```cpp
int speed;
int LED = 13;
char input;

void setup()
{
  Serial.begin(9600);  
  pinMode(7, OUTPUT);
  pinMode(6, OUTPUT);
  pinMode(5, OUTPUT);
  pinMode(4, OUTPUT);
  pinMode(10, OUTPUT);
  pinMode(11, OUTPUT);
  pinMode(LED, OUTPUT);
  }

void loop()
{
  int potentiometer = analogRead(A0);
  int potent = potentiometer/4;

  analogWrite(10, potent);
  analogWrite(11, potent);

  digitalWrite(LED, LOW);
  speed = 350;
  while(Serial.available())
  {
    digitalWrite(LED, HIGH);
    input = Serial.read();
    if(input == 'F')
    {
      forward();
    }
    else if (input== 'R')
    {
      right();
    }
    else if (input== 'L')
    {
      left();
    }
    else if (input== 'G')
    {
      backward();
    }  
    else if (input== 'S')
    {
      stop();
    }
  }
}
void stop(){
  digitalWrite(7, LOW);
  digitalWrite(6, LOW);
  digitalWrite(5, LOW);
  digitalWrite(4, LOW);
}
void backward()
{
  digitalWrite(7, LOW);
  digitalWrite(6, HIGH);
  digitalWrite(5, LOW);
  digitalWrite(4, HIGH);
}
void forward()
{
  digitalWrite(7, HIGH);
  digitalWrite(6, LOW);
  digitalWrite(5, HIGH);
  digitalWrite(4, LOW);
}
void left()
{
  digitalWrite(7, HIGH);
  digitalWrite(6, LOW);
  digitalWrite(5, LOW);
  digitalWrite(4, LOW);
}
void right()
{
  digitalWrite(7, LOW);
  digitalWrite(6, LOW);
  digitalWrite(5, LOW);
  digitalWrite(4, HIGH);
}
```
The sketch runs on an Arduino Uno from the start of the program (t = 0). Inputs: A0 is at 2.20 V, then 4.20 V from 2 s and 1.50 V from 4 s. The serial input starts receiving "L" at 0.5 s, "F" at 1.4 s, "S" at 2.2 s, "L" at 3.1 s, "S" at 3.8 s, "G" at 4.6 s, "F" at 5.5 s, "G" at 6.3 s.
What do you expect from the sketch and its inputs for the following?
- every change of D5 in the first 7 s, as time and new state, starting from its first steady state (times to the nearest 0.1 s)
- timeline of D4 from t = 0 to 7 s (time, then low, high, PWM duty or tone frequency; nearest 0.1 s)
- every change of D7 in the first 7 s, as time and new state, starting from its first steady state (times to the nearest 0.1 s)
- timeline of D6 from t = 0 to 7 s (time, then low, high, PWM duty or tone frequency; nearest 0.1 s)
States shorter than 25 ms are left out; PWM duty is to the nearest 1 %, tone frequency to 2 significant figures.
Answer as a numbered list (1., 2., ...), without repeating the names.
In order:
1. 0 s low; 1.4 s high; 2.2 s low; 5.5 s high; 6.3 s low
2. 0 s low; 4.6 s high; 5.5 s low; 6.3 s high
3. 0 s low; 0.5 s high; 2.2 s low; 3.1 s high; 3.8 s low; 5.5 s high; 6.3 s low
4. 0 s low; 4.6 s high; 5.5 s low; 6.3 s high
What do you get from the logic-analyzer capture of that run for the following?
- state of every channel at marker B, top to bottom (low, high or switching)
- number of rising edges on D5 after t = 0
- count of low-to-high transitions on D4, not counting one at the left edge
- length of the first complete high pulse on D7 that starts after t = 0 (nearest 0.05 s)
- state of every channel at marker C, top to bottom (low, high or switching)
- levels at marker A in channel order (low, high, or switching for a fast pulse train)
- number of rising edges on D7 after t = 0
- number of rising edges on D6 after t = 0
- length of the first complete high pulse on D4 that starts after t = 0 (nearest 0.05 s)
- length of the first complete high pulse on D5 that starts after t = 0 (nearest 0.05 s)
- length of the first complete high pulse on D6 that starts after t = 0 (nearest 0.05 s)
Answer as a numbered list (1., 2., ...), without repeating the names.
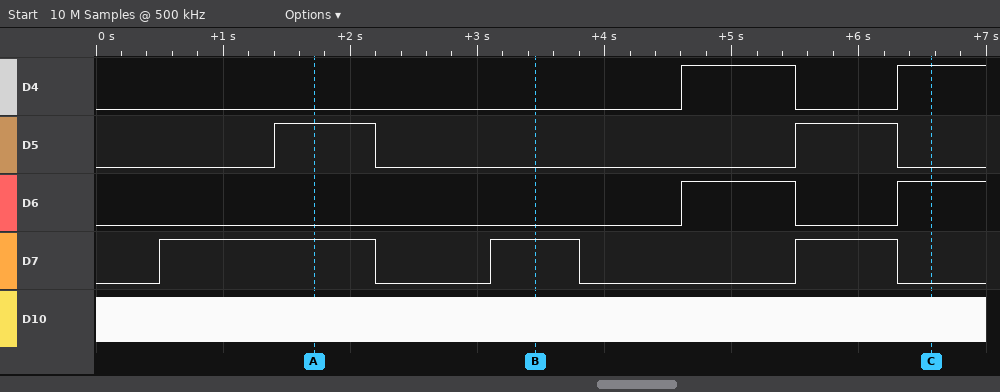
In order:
1. D4 low, D5 low, D6 low, D7 high, D10 switching
2. 2
3. 2
4. 1.70 s
5. D4 high, D5 low, D6 high, D7 low, D10 switching
6. D4 low, D5 high, D6 low, D7 high, D10 switching
7. 3
8. 2
9. 0.90 s
10. 0.80 s
11. 0.90 s
